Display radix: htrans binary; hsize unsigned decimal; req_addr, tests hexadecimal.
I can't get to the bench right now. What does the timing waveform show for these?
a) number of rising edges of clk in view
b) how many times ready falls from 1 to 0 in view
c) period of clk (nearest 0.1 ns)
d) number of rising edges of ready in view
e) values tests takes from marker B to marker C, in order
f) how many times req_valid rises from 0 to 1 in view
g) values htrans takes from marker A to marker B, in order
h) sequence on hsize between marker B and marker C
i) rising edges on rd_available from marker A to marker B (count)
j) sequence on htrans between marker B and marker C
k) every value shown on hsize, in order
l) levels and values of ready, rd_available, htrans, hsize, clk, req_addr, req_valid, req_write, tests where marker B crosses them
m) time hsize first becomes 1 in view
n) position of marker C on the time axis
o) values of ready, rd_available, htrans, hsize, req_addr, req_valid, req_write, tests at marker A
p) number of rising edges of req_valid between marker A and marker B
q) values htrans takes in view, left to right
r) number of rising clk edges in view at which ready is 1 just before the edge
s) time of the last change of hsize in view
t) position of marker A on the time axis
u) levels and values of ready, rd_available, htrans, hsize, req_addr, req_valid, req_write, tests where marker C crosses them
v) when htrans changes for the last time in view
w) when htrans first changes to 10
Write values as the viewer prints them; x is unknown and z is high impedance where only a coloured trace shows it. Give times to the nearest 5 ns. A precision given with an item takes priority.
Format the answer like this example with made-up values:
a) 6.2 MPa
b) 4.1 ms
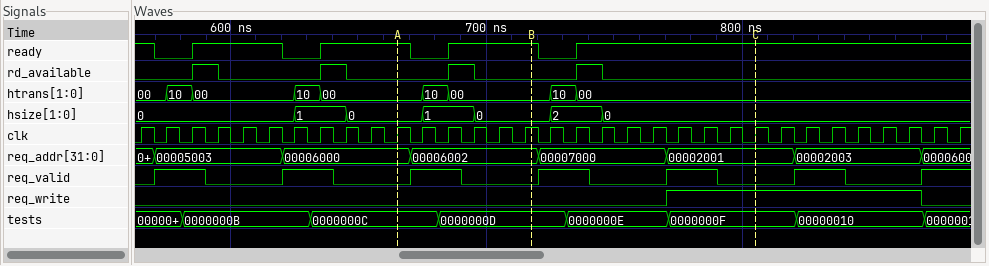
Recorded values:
a) 33
b) 4
c) 10 ns
d) 4
e) 0000000D, 0000000E, 0000000F
f) 7
g) 00, 10, 00
h) 0, 2, 0
i) 1
j) 00, 10, 00
k) 0, 1, 0, 1, 0, 2, 0
l) ready=1, rd_available=0, htrans=00, hsize=0, clk=1, req_addr=00006002, req_valid=0, req_write=0, tests=0000000D
m) 625 ns
n) 805 ns
o) ready=1, rd_available=0, htrans=00, hsize=0, req_addr=00006000, req_valid=0, req_write=0, tests=0000000C
p) 1
q) 00, 10, 00, 10, 00, 10, 00, 10, 00
r) 25
s) 745 ns
t) 665 ns
u) ready=1, rd_available=0, htrans=00, hsize=0, req_addr=00002001, req_valid=0, req_write=1, tests=0000000F
v) 735 ns
w) 575 ns
